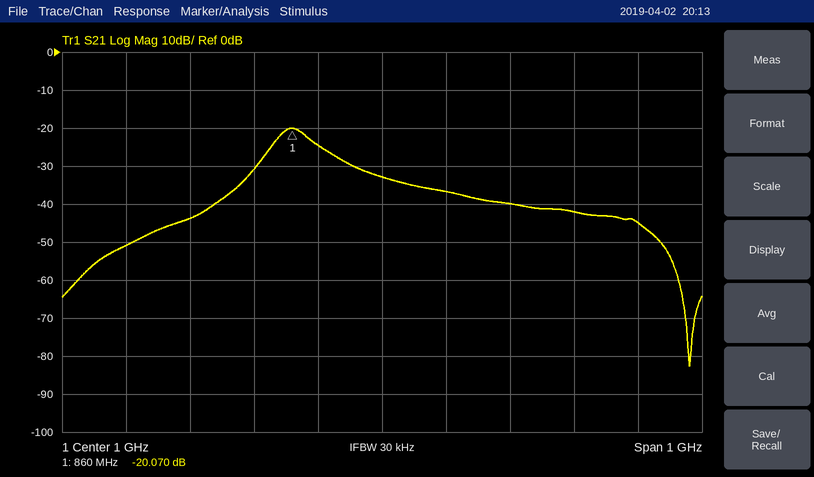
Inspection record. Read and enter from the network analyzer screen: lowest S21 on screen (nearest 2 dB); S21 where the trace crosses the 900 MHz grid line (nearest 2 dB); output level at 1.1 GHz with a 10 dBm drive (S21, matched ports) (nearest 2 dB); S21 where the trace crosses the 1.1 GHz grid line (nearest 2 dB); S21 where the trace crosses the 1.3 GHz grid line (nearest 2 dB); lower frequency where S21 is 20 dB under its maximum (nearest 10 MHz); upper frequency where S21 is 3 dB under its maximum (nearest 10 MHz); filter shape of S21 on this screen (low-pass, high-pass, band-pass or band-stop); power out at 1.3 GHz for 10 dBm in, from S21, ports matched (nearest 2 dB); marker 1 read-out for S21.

-82 dB
-24 dB
-26 dBm
-36 dB
-42 dB
740 MHz
890 MHz
band-pass
-32 dBm
-20.070 dB
